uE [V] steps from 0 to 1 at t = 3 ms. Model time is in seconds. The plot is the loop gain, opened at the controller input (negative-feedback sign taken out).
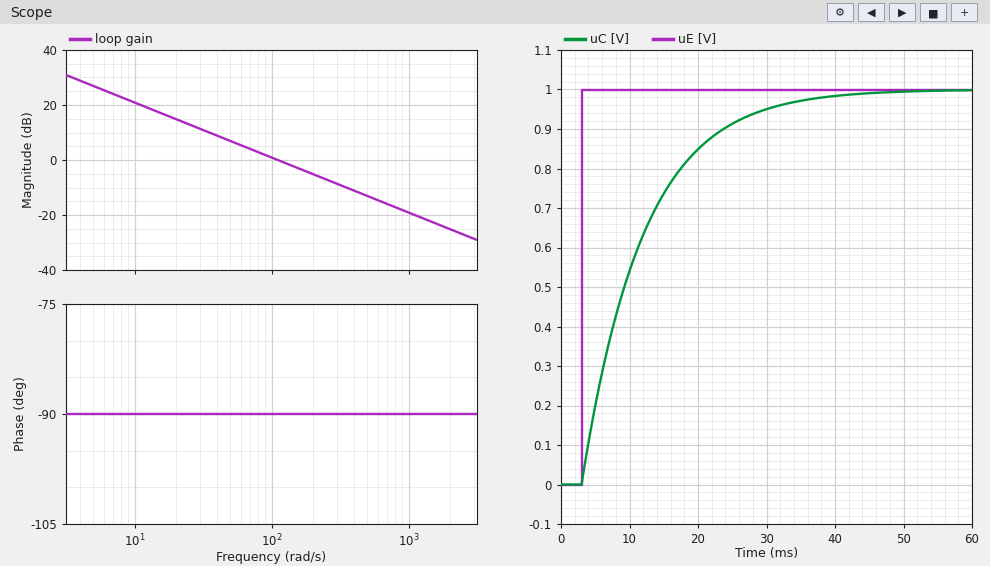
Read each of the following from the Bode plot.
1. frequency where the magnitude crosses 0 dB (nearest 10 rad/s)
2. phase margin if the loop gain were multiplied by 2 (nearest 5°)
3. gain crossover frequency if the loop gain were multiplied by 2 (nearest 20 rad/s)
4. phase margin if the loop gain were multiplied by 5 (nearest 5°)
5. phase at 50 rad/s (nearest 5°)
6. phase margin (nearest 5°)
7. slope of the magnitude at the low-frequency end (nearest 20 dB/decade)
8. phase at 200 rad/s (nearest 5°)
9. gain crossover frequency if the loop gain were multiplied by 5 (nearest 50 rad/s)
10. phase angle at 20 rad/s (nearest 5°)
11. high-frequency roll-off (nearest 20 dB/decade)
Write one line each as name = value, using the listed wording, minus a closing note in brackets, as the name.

frequency where the magnitude crosses 0 dB = 110 rad/s
phase margin if the loop gain were multiplied by 2 = 90°
gain crossover frequency if the loop gain were multiplied by 2 = 220 rad/s
phase margin if the loop gain were multiplied by 5 = 90°
phase at 50 rad/s = -90°
phase margin = 90°
slope of the magnitude at the low-frequency end = -20 dB/decade
phase at 200 rad/s = -90°
gain crossover frequency if the loop gain were multiplied by 5 = 550 rad/s
phase angle at 20 rad/s = -90°
high-frequency roll-off = -20 dB/decade
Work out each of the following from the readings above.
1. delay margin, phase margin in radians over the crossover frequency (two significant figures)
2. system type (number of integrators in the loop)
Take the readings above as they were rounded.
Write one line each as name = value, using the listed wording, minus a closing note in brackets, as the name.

delay margin, phase margin in radians over the crossover frequency = 0.014 s
system type = 1
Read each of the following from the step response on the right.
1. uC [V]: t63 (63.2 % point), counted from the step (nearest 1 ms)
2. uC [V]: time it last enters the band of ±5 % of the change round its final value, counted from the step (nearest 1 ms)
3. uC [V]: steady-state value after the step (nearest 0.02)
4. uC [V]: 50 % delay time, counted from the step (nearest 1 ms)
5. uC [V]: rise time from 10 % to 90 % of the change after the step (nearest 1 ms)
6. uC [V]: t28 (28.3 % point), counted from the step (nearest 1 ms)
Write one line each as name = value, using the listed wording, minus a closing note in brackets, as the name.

uC [V]: t63 (63.2 % point), counted from the step = 9 ms
uC [V]: time it last enters the band of ±5 % of the change round its final value, counted from the step = 27 ms
uC [V]: steady-state value after the step = 1.00
uC [V]: 50 % delay time, counted from the step = 6 ms
uC [V]: rise time from 10 % to 90 % of the change after the step = 20 ms
uC [V]: t28 (28.3 % point), counted from the step = 3 ms
